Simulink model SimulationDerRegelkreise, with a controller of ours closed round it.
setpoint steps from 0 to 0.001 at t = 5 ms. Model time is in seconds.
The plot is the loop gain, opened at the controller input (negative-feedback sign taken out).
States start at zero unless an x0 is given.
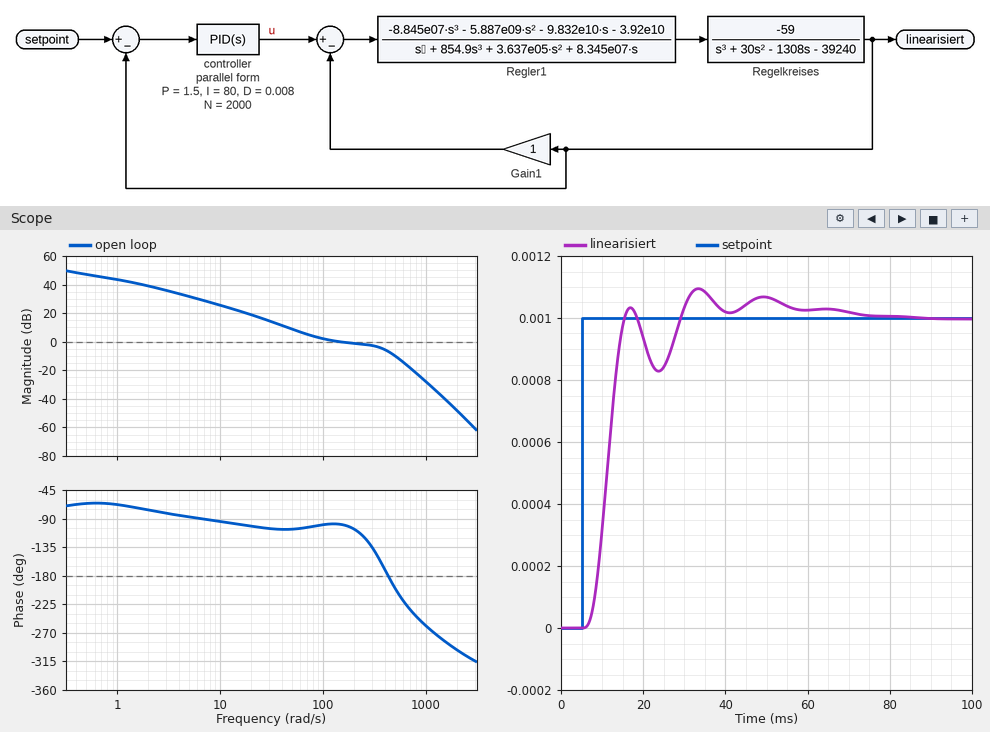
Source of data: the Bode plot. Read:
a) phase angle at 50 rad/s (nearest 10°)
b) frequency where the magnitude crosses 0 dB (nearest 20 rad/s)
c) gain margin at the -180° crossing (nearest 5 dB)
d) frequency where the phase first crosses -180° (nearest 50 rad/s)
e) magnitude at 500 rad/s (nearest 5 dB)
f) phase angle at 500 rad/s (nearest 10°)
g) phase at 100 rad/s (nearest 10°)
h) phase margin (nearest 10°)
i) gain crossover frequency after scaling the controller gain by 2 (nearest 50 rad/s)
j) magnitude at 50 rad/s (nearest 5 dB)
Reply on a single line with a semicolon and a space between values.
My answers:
-110°; 140 rad/s; 5 dB; 450 rad/s; -10 dB; -200°; -100°; 80°; 400 rad/s; 10 dB
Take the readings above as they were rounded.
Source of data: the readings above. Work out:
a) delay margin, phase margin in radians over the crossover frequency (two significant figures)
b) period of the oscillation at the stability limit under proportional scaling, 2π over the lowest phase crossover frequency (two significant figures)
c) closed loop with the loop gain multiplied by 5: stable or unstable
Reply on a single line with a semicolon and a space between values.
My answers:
0.0100 s; 0.014 s; unstable
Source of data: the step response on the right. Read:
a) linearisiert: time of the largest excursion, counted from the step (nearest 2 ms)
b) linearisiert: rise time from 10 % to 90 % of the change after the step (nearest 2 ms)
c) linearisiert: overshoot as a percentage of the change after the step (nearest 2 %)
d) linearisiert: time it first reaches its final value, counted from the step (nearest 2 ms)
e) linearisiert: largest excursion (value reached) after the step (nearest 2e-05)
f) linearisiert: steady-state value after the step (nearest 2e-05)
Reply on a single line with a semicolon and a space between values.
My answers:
28 ms; 6 ms; 10 %; 10 ms; 0.00110; 0.00100
